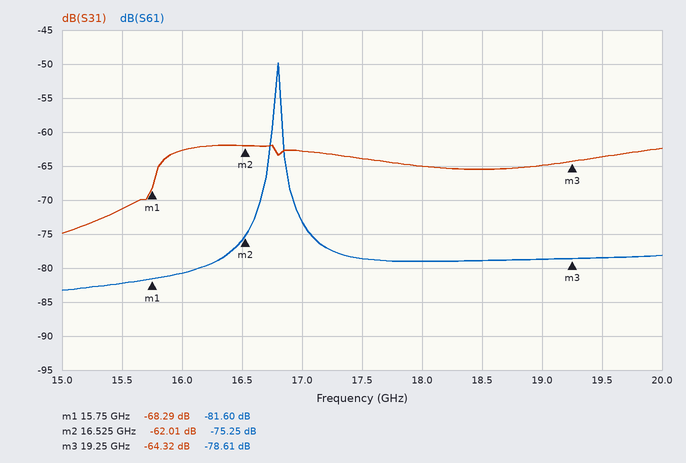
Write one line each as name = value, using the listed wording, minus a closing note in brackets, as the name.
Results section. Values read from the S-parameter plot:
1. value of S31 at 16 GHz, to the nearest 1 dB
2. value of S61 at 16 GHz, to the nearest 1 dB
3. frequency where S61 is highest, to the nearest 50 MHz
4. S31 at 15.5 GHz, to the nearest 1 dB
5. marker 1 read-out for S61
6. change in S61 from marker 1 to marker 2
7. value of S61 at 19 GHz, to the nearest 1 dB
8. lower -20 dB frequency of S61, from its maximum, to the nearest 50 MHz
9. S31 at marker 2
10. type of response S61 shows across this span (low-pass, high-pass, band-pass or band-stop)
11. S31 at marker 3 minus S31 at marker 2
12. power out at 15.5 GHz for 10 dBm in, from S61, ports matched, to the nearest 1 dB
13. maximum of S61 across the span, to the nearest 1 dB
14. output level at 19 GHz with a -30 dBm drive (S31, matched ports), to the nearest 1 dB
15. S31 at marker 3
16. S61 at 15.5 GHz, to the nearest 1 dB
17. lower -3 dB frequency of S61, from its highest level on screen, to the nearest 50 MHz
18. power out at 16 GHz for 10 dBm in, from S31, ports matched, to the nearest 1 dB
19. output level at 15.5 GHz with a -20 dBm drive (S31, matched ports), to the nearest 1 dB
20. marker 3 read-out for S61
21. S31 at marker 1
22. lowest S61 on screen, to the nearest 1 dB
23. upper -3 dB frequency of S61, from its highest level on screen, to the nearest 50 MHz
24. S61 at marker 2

value of S31 at 16 GHz, to the nearest 1 dB = -63 dB
value of S61 at 16 GHz, to the nearest 1 dB = -81 dB
frequency where S61 is highest, to the nearest 50 MHz = 16.80 GHz
S31 at 15.5 GHz, to the nearest 1 dB = -71 dB
marker 1 read-out for S61 = -81.60 dB
change in S61 from marker 1 to marker 2 = 6.35 dB
value of S61 at 19 GHz, to the nearest 1 dB = -79 dB
lower -20 dB frequency of S61, from its maximum, to the nearest 50 MHz = 16.65 GHz
S31 at marker 2 = -62.01 dB
type of response S61 shows across this span = band-pass
S31 at marker 3 minus S31 at marker 2 = -2.31 dB
power out at 15.5 GHz for 10 dBm in, from S61, ports matched, to the nearest 1 dB = -72 dBm
maximum of S61 across the span, to the nearest 1 dB = -50 dB
output level at 19 GHz with a -30 dBm drive (S31, matched ports), to the nearest 1 dB = -95 dBm
S31 at marker 3 = -64.32 dB
S61 at 15.5 GHz, to the nearest 1 dB = -82 dB
lower -3 dB frequency of S61, from its highest level on screen, to the nearest 50 MHz = 16.80 GHz
power out at 16 GHz for 10 dBm in, from S31, ports matched, to the nearest 1 dB = -53 dBm
output level at 15.5 GHz with a -20 dBm drive (S31, matched ports), to the nearest 1 dB = -91 dBm
marker 3 read-out for S61 = -78.61 dB
S31 at marker 1 = -68.29 dB
lowest S61 on screen, to the nearest 1 dB = -83 dB
upper -3 dB frequency of S61, from its highest level on screen, to the nearest 50 MHz = 16.80 GHz
S61 at marker 2 = -75.25 dB
